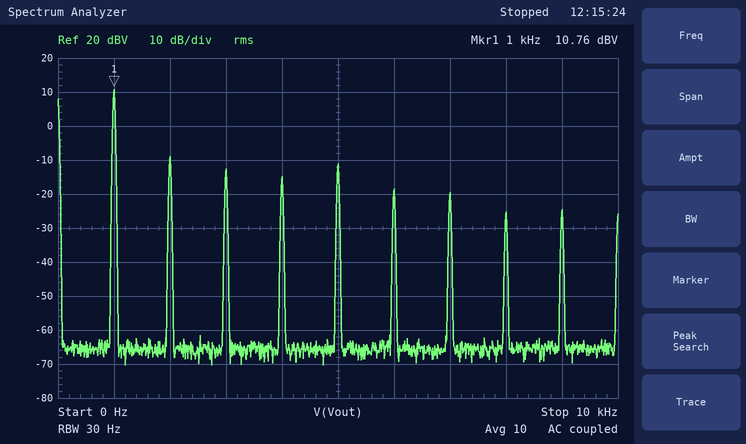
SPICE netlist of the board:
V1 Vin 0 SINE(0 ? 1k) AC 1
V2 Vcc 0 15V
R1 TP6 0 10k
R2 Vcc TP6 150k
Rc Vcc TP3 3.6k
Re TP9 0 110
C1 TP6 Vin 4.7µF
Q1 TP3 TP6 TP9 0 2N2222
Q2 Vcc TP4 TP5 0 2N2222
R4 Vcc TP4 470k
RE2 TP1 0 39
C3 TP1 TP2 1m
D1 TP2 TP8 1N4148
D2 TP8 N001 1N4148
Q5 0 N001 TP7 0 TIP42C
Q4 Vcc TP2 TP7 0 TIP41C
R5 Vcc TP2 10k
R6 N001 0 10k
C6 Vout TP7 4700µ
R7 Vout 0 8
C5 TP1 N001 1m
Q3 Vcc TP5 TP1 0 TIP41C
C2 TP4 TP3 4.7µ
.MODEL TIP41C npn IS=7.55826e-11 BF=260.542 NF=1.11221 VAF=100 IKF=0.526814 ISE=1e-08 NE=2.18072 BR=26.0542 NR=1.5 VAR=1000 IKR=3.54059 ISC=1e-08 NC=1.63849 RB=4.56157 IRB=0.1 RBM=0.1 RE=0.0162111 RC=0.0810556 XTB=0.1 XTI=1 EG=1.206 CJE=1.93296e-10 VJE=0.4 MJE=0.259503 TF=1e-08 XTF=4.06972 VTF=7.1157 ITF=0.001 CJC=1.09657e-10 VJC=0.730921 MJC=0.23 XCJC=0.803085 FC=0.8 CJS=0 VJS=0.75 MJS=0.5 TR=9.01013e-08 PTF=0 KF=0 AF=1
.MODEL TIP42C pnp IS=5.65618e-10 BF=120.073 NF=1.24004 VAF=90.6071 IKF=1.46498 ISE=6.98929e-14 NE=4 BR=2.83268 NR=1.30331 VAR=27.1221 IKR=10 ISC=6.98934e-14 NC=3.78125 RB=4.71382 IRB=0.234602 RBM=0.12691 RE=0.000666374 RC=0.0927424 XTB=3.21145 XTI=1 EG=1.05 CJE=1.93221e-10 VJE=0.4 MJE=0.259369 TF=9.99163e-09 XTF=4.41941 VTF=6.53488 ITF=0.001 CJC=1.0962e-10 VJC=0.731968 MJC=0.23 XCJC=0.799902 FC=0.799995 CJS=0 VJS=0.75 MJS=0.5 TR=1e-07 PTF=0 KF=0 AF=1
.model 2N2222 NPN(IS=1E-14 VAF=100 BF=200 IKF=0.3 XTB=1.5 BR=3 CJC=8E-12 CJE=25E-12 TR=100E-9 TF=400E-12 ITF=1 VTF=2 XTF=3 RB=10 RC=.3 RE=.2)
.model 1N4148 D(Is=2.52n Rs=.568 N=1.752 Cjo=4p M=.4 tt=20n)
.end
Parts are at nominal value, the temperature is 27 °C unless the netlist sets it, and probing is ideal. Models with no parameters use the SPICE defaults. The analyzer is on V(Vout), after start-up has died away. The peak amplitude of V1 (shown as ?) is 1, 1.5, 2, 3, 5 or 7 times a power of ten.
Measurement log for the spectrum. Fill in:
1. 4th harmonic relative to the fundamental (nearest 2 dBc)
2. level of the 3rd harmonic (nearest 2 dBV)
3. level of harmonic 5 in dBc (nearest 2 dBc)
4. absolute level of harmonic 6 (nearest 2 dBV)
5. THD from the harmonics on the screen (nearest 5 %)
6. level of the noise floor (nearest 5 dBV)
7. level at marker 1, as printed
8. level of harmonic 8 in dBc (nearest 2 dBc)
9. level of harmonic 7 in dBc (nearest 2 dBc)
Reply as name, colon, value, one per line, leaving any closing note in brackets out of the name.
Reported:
4th harmonic relative to the fundamental: -26 dBc
level of the 3rd harmonic: -12 dBV
level of harmonic 5 in dBc: -22 dBc
absolute level of harmonic 6: -18 dBV
THD from the harmonics on the screen: 15 %
level of the noise floor: -65 dBV
level at marker 1, as printed: 10.76 dBV
level of harmonic 8 in dBc: -36 dBc
level of harmonic 7 in dBc: -30 dBc
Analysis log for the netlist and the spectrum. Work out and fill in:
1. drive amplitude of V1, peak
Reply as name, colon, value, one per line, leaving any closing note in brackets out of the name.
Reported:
drive amplitude of V1, peak: 300 mV
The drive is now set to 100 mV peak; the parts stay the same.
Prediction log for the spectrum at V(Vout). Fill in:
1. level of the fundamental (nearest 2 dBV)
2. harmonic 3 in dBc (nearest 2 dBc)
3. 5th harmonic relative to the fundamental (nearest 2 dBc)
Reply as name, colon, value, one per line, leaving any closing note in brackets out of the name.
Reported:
level of the fundamental: 4 dBV
harmonic 3 in dBc: -28 dBc
5th harmonic relative to the fundamental: -34 dBc
